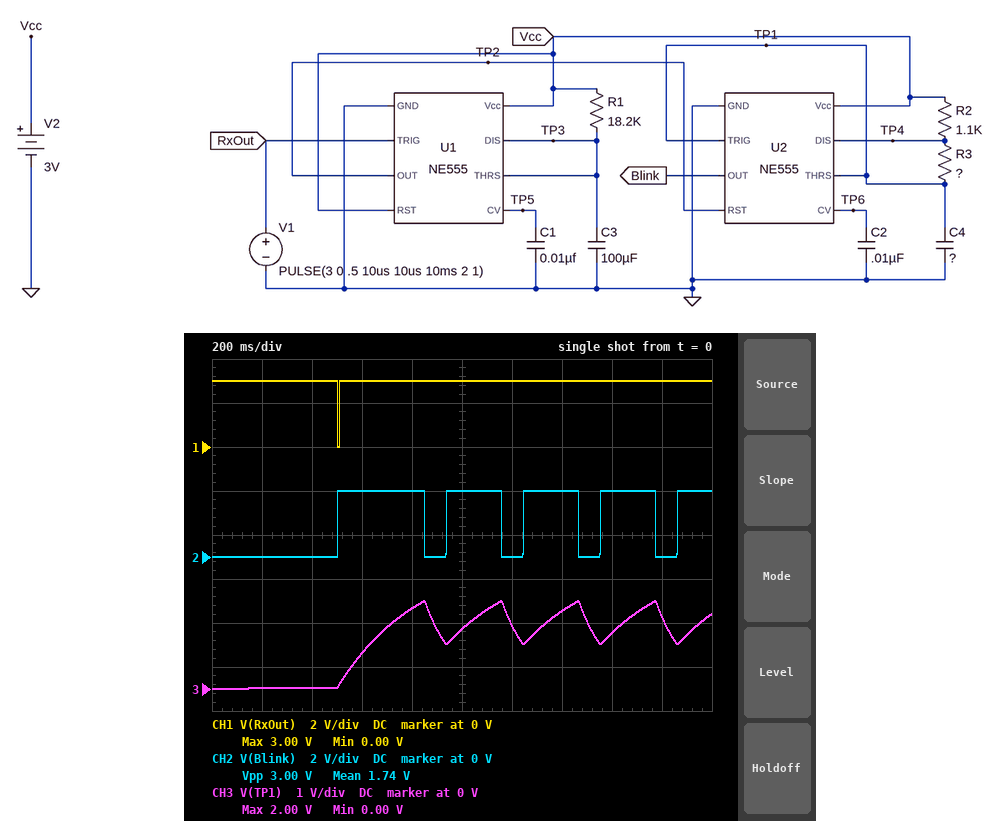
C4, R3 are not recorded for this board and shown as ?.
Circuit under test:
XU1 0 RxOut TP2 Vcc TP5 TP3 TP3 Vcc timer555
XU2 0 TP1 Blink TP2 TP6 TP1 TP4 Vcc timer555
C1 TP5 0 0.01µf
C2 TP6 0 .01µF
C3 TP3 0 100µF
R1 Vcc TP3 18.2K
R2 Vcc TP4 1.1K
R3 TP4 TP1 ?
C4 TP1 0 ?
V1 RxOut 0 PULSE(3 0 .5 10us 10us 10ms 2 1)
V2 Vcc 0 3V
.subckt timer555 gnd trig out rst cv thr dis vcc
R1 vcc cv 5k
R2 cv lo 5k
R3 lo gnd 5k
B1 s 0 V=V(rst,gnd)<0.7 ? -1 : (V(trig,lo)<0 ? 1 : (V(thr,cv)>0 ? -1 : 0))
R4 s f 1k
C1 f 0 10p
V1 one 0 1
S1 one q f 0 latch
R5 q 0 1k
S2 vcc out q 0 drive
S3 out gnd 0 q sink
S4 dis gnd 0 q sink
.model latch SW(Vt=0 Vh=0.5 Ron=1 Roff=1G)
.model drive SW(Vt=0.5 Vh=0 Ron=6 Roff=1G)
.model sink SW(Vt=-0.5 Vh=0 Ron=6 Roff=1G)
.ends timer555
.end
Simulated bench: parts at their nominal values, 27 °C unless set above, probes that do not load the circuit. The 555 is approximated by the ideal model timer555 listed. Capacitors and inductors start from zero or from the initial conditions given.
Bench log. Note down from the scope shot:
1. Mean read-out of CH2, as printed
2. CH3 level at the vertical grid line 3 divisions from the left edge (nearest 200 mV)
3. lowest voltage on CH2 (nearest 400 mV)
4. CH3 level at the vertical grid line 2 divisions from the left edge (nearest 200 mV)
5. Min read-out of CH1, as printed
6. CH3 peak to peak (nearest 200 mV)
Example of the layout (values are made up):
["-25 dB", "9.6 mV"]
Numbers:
["1.74 V", "800 mV", "0 V", "0 V", "0.00 V", "2.0 V"]
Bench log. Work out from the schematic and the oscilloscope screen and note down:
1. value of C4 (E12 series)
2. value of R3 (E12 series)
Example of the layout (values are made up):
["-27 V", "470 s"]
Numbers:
["180 µF", "680 Ω"]
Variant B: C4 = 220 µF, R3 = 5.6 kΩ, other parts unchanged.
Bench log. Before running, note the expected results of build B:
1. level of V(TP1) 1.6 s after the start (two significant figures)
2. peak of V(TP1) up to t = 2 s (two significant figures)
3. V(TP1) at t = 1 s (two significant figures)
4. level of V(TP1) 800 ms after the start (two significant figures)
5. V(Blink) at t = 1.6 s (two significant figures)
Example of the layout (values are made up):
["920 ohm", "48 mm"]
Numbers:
["1.6 V", "1.9 V", "870 mV", "560 mV", "3.0 V"]
